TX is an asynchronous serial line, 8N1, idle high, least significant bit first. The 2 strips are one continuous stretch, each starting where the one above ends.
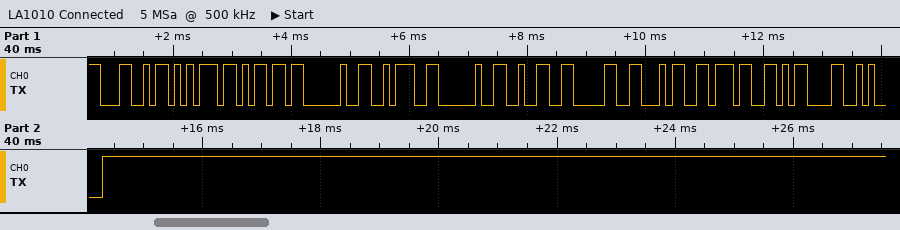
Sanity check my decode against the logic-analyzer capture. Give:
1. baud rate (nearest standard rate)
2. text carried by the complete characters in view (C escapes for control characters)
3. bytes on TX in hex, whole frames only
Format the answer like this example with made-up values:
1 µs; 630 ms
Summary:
9600 baud; "Lum : 2047\r\n"; 0x4C 0x75 0x6D 0x20 0x3A 0x20 0x32 0x30 0x34 0x37 0x0D 0x0A
